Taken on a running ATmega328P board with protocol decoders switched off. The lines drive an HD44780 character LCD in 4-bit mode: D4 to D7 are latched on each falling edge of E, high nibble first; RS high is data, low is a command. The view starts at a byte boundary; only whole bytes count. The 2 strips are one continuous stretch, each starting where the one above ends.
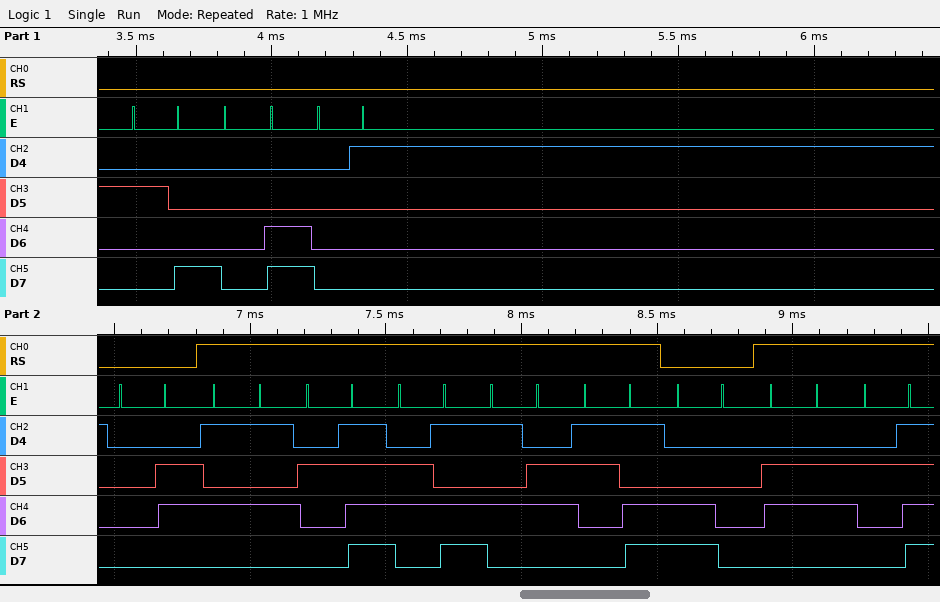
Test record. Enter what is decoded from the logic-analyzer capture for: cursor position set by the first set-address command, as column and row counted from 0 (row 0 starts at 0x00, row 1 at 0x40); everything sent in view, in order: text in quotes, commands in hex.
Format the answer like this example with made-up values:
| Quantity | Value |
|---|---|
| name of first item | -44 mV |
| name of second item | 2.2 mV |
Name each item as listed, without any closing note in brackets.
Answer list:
| Quantity | Value |
|---|---|
| cursor position set by the first set-address command, as column and row counted from 0 | column 0, row 1 |
| everything sent in view, in order: text in quotes, commands in hex | 0x28 0x0C 0x01 0x06 "U/mV=" 0xC0 "f/" |
